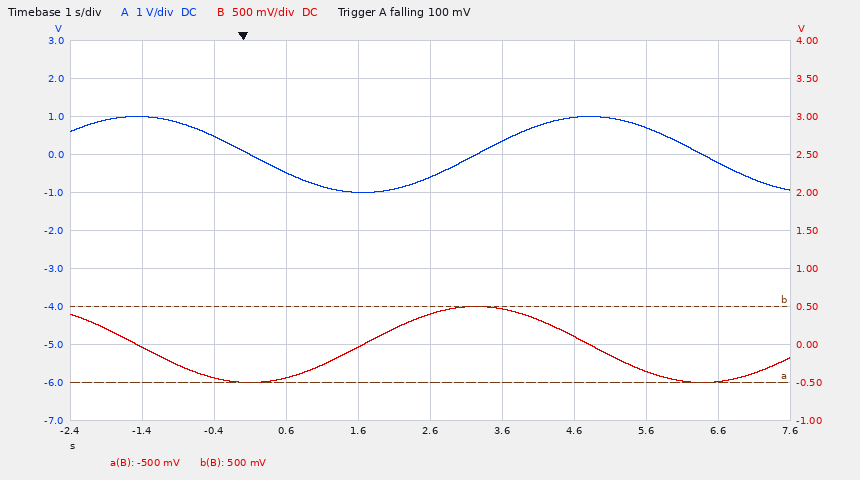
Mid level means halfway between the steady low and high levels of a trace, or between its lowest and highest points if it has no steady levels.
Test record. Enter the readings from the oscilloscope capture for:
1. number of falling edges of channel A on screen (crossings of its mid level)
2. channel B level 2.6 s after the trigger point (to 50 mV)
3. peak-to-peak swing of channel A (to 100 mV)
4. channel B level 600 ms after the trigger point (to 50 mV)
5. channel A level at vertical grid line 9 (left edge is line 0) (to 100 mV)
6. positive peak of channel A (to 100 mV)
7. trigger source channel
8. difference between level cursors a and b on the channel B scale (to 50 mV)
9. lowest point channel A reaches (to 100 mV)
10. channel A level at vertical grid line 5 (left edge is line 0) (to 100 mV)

2
400 mV
2.0 V
-450 mV
-200 mV
1.0 V
channel A
1.00 V
-1.0 V
-600 mV
